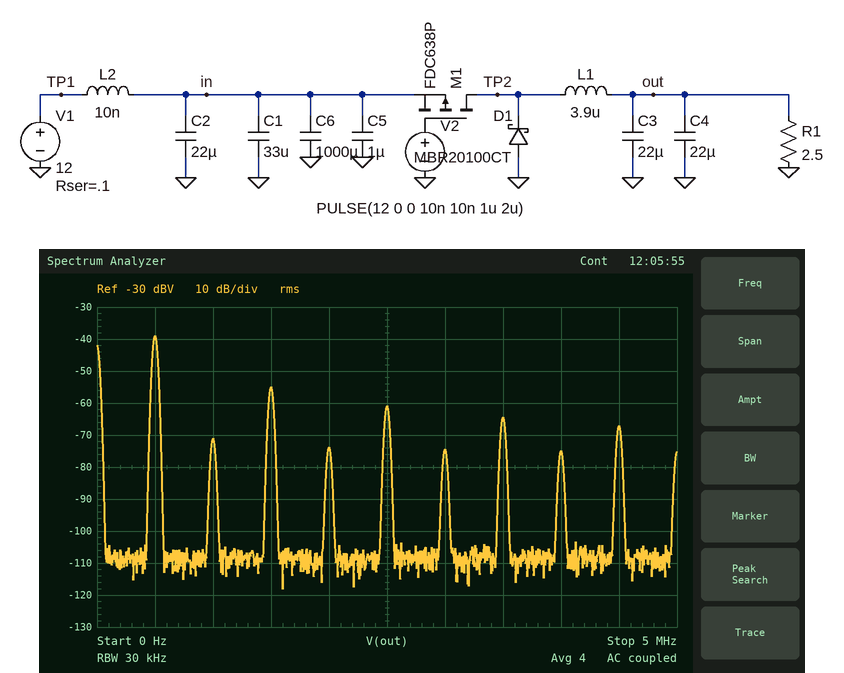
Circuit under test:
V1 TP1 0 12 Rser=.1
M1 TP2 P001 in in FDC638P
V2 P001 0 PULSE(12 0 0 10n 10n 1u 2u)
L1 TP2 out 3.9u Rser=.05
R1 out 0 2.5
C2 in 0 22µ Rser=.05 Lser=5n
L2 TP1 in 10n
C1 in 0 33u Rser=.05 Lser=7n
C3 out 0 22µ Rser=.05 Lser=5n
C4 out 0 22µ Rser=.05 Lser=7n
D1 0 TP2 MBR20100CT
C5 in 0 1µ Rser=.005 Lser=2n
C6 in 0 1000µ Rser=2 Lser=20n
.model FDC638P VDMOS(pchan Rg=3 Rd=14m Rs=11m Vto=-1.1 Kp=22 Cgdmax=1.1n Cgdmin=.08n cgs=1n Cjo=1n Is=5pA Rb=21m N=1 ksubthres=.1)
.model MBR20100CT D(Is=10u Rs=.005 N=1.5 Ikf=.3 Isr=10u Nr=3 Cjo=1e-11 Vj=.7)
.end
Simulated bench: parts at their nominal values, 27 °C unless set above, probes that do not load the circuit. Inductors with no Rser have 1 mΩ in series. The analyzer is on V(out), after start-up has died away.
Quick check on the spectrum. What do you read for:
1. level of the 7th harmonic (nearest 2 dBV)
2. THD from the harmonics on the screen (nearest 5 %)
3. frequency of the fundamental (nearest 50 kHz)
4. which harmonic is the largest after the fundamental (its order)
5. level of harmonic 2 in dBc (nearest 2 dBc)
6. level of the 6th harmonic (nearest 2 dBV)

-64 dBV
20 %
500 kHz
3
-32 dBc
-74 dBV
